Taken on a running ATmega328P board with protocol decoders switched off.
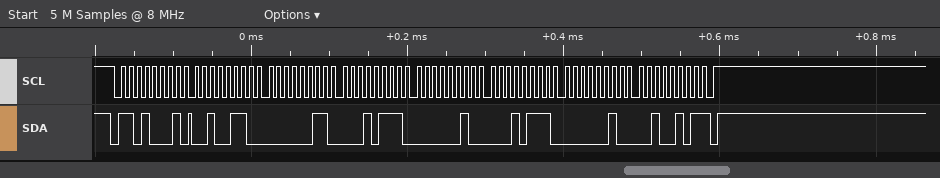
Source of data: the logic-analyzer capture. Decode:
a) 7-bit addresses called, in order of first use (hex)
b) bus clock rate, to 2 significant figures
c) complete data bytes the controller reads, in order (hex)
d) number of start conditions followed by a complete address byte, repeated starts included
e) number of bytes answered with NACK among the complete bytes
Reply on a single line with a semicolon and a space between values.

0x68; 100 kHz; 26 03 17 02 17 02 25; 1; 1
